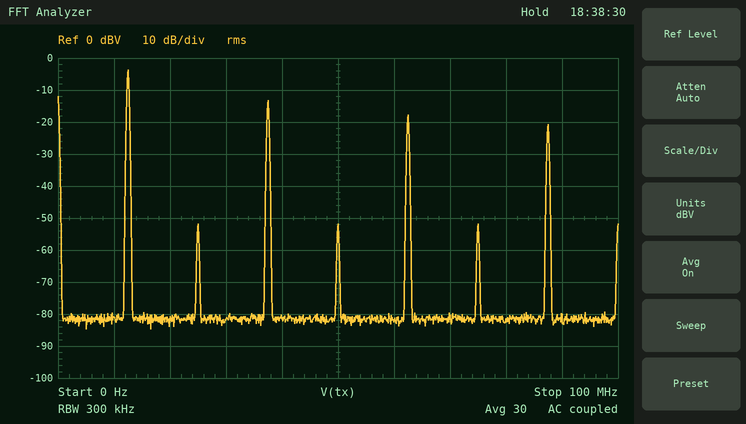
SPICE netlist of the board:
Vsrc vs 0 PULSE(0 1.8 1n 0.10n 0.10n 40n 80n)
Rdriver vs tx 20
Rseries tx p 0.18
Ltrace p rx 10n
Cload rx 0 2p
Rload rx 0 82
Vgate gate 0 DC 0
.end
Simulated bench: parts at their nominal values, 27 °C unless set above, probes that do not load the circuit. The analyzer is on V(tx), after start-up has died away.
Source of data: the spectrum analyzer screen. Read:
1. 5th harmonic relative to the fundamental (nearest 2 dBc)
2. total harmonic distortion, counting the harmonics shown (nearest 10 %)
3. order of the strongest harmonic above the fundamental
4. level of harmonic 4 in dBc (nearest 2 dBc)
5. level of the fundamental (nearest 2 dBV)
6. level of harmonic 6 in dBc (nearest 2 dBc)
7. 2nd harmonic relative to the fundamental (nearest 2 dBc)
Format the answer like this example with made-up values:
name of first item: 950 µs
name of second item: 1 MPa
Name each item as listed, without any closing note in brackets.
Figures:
5th harmonic relative to the fundamental: -14 dBc
total harmonic distortion, counting the harmonics shown: 40 %
order of the strongest harmonic above the fundamental: 3
level of harmonic 4 in dBc: -48 dBc
level of the fundamental: -4 dBV
level of harmonic 6 in dBc: -48 dBc
2nd harmonic relative to the fundamental: -48 dBc
